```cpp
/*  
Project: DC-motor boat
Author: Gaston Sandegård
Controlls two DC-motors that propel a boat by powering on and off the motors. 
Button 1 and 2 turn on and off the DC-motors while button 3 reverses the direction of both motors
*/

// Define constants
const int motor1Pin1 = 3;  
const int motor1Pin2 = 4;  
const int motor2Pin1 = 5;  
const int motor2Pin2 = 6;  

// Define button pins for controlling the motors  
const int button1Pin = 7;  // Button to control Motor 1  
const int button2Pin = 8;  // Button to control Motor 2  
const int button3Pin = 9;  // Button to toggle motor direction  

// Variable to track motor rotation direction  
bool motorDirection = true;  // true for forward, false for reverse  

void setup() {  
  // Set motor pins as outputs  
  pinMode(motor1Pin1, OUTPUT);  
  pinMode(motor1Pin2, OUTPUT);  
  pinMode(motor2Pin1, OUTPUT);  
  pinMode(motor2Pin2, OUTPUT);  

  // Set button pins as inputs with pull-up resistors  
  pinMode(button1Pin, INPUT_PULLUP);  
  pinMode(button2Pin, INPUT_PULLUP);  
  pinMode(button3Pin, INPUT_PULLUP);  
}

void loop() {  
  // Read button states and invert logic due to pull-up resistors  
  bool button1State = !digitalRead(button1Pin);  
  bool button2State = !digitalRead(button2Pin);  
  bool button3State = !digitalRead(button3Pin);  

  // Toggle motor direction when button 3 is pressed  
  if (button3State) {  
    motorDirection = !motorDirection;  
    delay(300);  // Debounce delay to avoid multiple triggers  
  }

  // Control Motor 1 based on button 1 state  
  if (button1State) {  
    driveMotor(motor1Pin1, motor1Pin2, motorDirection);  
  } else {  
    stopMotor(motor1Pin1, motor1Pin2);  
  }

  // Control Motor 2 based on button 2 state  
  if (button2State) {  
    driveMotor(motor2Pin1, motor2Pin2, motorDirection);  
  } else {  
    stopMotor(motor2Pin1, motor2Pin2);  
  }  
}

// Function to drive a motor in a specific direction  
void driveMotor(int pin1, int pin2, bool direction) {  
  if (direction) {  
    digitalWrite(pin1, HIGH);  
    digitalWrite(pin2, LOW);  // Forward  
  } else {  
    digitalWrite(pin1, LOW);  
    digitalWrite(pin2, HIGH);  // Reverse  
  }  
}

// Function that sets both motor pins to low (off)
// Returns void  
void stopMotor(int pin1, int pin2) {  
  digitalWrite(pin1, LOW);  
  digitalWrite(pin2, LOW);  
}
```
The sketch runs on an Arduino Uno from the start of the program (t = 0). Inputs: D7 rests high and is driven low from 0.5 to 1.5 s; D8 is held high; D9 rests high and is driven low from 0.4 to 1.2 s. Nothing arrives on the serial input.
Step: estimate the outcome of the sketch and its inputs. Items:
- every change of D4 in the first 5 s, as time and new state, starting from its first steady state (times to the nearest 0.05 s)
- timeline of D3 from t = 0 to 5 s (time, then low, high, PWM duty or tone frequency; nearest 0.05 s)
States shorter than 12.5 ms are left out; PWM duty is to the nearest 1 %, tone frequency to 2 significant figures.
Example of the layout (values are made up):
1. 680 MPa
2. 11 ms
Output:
1. 0 s low; 1.3 s high; 1.5 s low
2. 0 s low; 1 s high; 1.3 s low
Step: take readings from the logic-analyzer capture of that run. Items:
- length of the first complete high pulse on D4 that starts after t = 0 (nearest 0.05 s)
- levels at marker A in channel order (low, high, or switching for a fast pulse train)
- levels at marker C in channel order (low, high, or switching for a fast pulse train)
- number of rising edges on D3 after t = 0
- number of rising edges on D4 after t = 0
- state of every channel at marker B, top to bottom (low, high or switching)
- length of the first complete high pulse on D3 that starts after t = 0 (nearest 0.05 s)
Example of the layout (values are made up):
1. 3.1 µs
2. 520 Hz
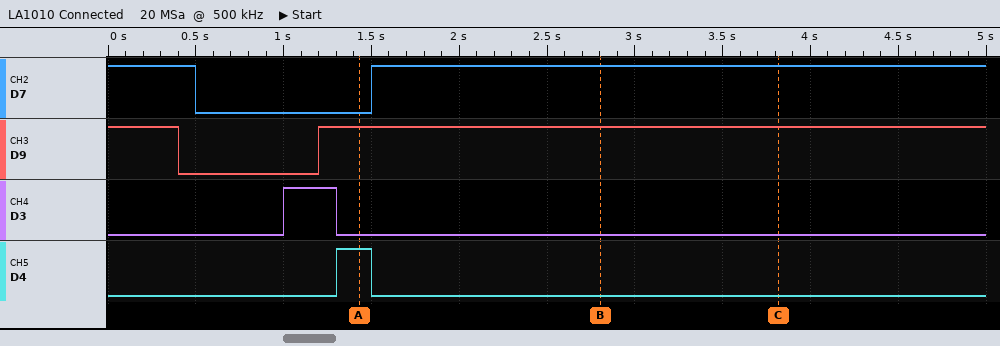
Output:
1. 0.20 s
2. D7 low, D9 high, D3 low, D4 high
3. D7 high, D9 high, D3 low, D4 low
4. 1
5. 1
6. D7 high, D9 high, D3 low, D4 low
7. 0.30 s
